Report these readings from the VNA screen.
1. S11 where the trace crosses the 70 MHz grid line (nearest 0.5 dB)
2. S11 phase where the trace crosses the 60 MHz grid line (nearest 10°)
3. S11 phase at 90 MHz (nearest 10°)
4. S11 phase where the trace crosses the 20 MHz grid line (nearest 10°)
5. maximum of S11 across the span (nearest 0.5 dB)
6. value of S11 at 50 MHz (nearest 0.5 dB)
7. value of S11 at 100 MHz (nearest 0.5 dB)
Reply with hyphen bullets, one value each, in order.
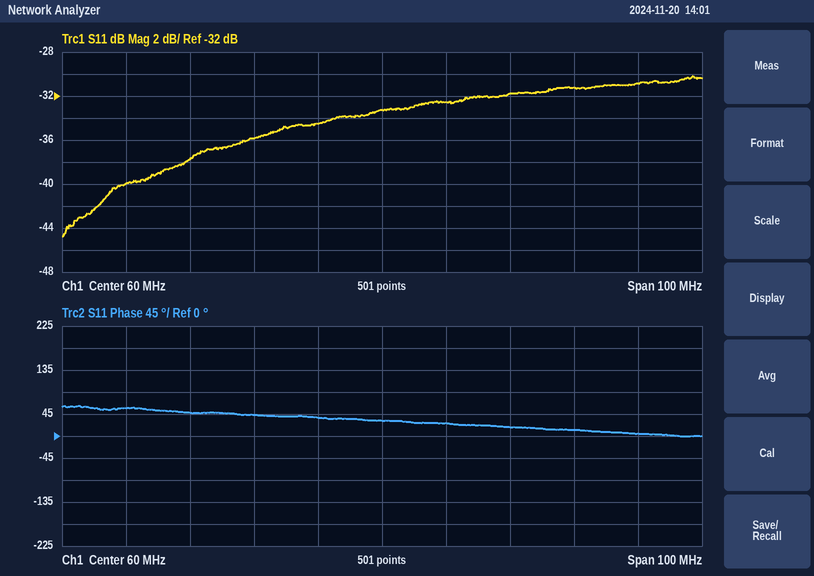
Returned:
- -32.5 dB
- 30°
- 10°
- 60°
- -30.0 dB
- -34.5 dB
- -31.0 dB
